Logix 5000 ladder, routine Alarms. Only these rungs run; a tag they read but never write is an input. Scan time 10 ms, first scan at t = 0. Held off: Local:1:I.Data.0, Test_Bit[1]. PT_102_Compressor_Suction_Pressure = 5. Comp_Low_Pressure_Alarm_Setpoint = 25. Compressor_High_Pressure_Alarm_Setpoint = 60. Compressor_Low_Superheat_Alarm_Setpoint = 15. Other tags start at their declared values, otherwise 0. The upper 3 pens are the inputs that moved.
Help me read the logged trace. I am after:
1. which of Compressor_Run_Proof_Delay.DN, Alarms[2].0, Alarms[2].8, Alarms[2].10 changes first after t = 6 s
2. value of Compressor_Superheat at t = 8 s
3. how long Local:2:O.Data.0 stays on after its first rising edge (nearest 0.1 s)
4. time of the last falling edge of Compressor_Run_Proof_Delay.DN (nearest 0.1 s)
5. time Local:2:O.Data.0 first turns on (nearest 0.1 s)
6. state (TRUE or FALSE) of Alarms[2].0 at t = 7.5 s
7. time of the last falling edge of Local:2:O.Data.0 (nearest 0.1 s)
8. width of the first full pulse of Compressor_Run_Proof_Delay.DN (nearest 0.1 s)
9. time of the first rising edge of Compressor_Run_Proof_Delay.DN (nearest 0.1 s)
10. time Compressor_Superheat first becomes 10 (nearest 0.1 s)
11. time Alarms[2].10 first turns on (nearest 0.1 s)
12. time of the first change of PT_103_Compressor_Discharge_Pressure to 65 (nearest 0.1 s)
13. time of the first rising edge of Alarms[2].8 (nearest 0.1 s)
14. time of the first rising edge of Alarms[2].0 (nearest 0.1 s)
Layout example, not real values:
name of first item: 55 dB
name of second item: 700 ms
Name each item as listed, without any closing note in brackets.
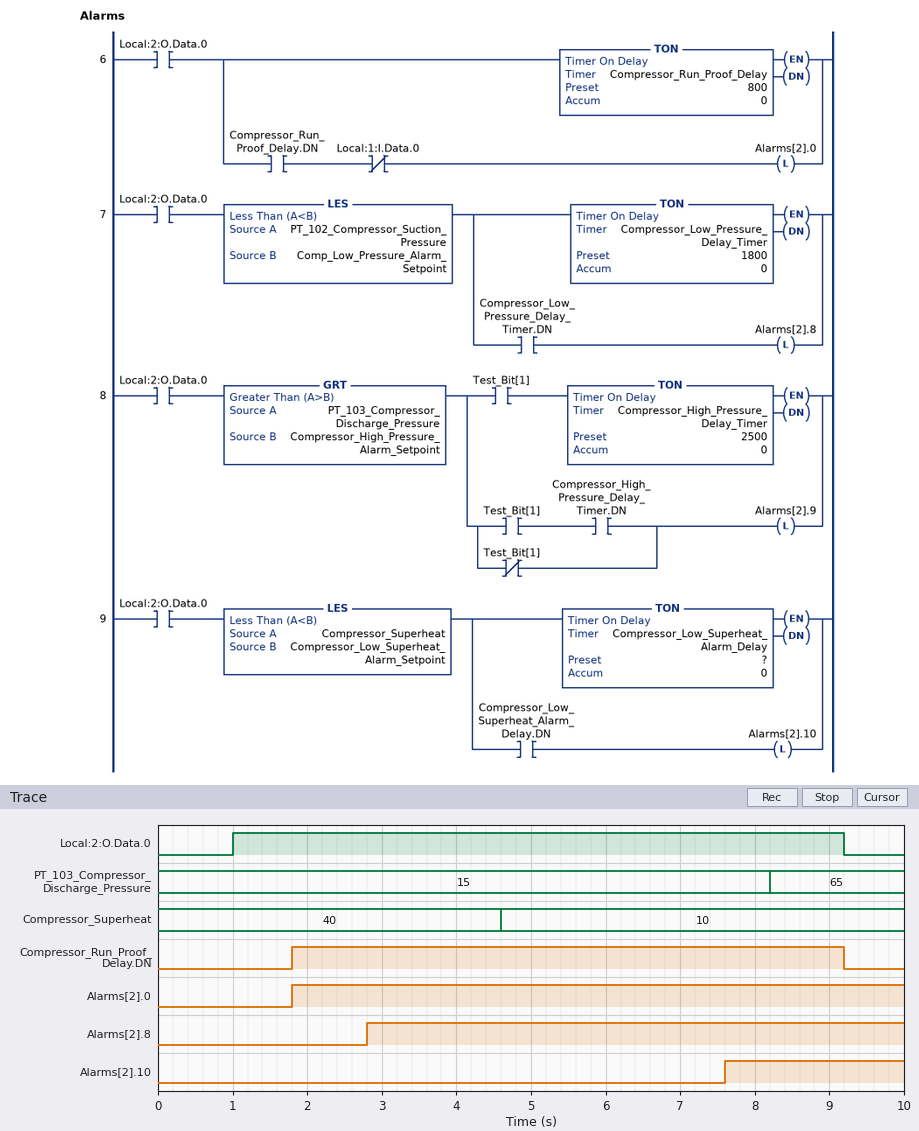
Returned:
which of Compressor_Run_Proof_Delay.DN, Alarms[2].0, Alarms[2].8, Alarms[2].10 changes first after t = 6 s: Alarms[2].10
value of Compressor_Superheat at t = 8 s: 10
how long Local:2:O.Data.0 stays on after its first rising edge: 8.2 s
time of the last falling edge of Compressor_Run_Proof_Delay.DN: 9.2 s
time Local:2:O.Data.0 first turns on: 1.0 s
state (TRUE or FALSE) of Alarms[2].0 at t = 7.5 s: TRUE
time of the last falling edge of Local:2:O.Data.0: 9.2 s
width of the first full pulse of Compressor_Run_Proof_Delay.DN: 7.4 s
time of the first rising edge of Compressor_Run_Proof_Delay.DN: 1.8 s
time Compressor_Superheat first becomes 10: 4.6 s
time Alarms[2].10 first turns on: 7.6 s
time of the first change of PT_103_Compressor_Discharge_Pressure to 65: 8.2 s
time of the first rising edge of Alarms[2].8: 2.8 s
time of the first rising edge of Alarms[2].0: 1.8 s
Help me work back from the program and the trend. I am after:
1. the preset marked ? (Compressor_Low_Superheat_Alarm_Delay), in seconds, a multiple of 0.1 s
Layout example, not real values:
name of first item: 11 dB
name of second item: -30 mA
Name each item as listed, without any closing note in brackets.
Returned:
the preset marked ? (Compressor_Low_Superheat_Alarm_Delay), in seconds, a multiple of 0.1 s: 3.0 s
